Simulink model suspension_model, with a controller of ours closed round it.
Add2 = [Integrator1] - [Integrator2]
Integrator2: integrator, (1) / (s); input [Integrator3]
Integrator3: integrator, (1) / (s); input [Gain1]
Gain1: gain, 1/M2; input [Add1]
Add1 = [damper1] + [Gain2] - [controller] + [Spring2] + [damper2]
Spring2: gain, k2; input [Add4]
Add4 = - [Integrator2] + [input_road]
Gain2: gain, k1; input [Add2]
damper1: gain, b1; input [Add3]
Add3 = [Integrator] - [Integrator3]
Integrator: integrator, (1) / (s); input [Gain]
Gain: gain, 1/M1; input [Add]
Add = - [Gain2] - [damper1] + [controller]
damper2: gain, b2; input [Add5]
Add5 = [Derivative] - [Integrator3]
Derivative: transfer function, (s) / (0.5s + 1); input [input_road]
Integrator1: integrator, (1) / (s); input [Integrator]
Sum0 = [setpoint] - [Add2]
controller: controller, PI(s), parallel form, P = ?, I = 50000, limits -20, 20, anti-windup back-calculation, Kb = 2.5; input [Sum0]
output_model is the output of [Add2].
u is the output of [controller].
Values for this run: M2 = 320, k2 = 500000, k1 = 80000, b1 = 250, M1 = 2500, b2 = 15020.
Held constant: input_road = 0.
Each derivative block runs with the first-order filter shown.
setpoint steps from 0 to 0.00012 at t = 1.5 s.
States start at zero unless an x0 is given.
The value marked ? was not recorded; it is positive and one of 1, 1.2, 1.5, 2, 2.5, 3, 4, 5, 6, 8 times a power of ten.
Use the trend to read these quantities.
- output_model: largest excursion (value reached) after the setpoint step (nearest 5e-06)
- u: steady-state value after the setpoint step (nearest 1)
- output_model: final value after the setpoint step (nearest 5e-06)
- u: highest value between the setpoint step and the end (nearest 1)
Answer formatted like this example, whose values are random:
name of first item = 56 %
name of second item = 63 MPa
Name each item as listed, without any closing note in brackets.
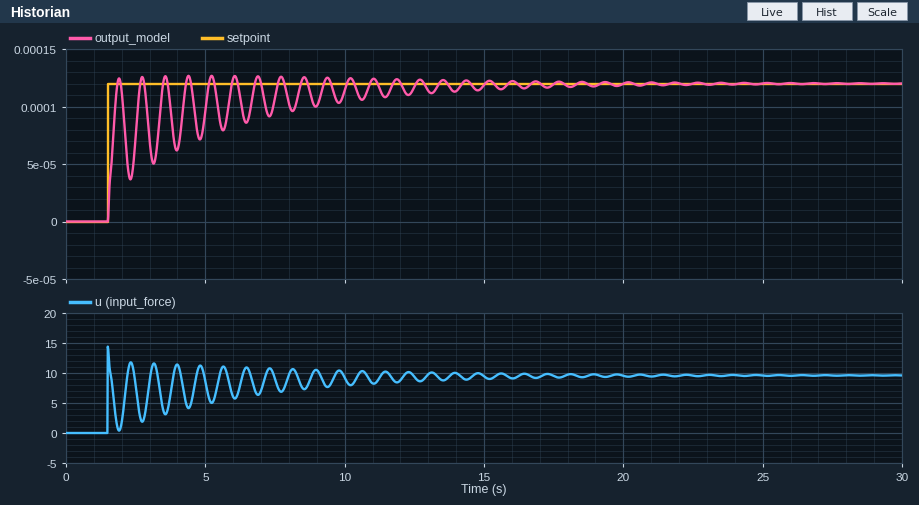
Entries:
output_model: largest excursion (value reached) after the setpoint step = 0.000125
u: steady-state value after the setpoint step = 10
output_model: final value after the setpoint step = 0.000120
u: highest value between the setpoint step and the end = 14
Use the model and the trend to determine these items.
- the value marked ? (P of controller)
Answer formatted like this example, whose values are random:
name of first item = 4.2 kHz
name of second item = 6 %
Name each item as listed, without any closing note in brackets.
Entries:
the value marked ? = 120000
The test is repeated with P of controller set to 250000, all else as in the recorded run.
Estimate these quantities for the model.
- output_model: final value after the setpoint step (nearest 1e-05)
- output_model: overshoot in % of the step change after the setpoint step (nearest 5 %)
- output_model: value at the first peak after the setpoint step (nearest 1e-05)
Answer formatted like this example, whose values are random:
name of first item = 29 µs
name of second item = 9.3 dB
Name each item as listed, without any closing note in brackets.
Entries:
output_model: final value after the setpoint step = 0.00012
output_model: overshoot in % of the step change after the setpoint step = 15 %
output_model: value at the first peak after the setpoint step = 0.00014
